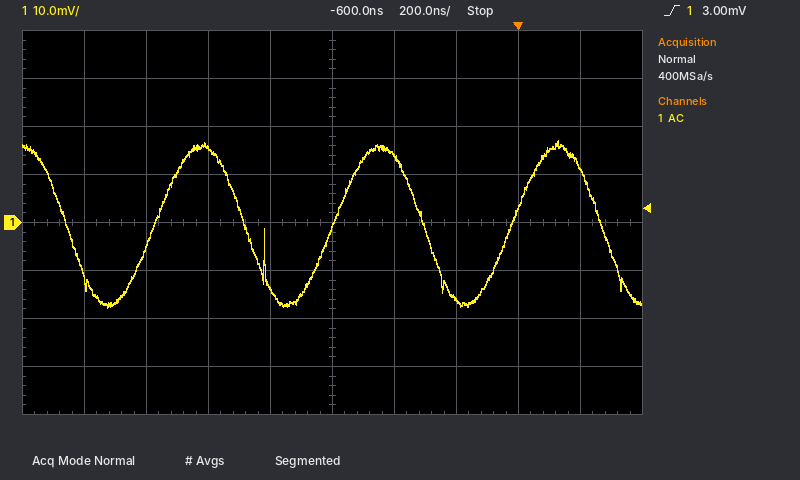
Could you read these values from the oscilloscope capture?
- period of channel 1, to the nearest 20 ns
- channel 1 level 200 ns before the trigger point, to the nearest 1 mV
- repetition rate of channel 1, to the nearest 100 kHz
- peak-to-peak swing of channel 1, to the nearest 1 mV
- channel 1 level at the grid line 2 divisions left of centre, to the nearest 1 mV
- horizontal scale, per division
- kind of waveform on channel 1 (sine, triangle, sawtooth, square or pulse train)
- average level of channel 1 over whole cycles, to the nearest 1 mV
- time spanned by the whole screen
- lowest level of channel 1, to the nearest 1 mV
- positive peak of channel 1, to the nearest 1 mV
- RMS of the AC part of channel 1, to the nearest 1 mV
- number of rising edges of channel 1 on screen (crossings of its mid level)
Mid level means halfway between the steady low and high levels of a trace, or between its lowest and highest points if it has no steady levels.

580 ns
-16 mV
1.7 MHz
35 mV
16 mV
200 ns
sine
0 mV
2 µs
-18 mV
17 mV
12 mV
3
